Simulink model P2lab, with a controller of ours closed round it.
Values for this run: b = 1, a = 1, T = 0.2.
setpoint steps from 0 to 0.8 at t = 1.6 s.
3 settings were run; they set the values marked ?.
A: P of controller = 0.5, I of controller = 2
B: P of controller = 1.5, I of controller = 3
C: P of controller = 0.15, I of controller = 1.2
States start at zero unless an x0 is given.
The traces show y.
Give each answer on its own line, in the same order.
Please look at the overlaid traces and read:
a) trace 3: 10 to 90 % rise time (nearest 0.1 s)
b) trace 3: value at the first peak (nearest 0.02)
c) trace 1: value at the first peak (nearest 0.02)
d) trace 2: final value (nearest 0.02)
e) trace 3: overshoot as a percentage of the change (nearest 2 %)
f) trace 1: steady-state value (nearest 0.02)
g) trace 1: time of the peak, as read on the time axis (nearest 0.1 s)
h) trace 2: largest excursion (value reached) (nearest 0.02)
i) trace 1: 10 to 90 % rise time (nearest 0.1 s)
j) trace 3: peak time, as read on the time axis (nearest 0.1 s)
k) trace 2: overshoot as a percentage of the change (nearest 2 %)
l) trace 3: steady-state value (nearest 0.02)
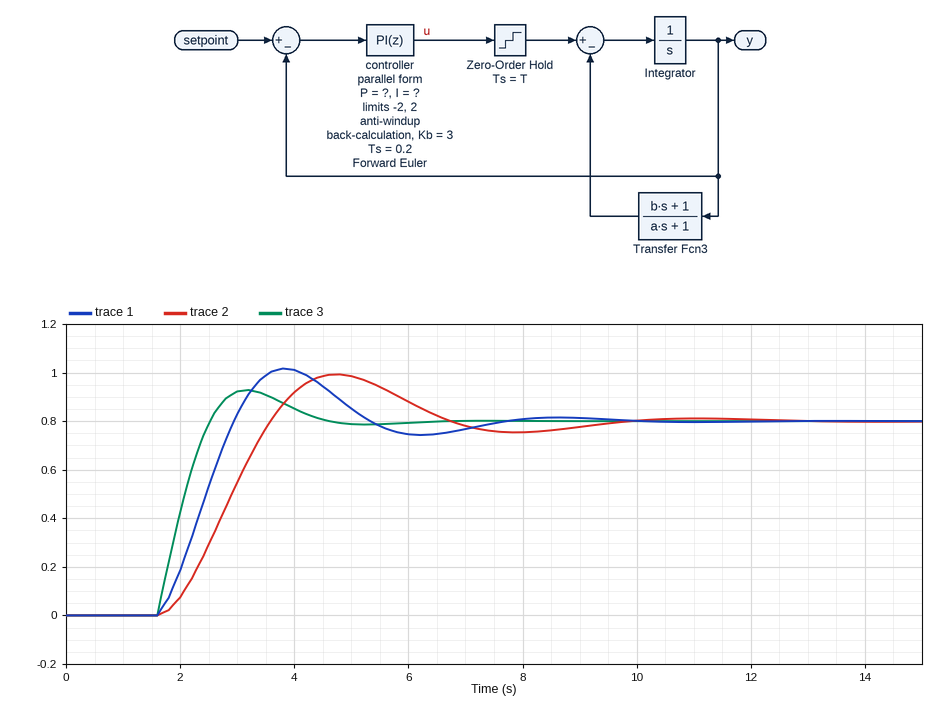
0.7 s
0.92
1.02
0.80
16 %
0.80
3.8 s
1.00
1.0 s
3.2 s
24 %
0.80
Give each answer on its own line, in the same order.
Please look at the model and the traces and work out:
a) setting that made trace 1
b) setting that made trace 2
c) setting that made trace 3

A
C
B
